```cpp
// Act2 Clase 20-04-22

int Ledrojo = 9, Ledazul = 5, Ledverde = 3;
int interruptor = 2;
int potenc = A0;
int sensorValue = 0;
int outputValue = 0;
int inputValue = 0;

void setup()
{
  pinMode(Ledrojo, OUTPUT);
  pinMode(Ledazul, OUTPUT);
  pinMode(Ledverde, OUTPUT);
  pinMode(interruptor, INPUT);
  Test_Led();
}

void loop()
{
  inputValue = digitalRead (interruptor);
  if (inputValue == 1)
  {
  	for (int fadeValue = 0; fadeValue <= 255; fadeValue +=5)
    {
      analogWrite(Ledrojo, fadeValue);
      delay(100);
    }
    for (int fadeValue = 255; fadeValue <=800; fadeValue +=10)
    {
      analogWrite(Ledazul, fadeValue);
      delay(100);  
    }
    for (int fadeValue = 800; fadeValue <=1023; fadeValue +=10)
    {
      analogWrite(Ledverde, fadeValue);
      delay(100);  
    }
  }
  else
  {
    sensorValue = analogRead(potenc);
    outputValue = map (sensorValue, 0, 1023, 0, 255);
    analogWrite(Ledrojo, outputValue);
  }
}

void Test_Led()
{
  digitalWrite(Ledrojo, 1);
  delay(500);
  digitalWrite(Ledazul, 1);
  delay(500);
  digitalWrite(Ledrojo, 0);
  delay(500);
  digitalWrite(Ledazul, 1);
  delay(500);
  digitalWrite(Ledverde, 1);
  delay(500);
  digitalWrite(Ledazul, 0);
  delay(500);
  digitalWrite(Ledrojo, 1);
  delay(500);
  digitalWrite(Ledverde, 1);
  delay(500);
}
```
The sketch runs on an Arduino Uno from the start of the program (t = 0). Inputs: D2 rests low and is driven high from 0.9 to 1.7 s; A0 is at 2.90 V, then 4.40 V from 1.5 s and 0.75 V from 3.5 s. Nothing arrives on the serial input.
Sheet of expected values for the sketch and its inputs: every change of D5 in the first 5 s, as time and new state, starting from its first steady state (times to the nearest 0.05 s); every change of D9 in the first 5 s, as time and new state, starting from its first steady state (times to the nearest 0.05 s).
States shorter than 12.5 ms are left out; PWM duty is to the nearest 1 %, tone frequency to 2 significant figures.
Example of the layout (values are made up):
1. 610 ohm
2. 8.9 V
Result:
1. 0 s low; 0.5 s high; 2.5 s low
2. 0 s high; 1 s low; 3 s high; 4 s PWM 15 %
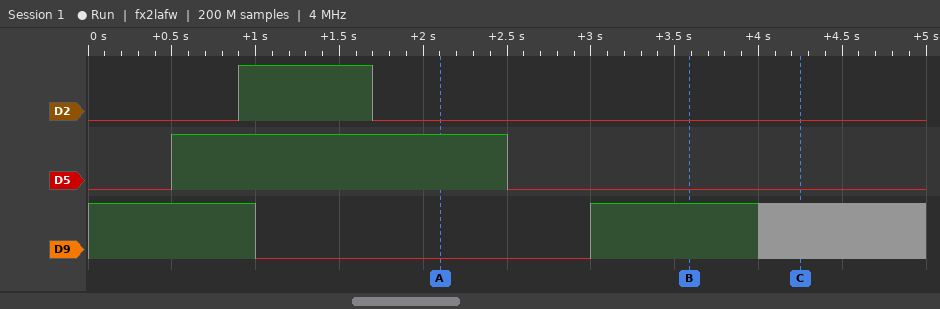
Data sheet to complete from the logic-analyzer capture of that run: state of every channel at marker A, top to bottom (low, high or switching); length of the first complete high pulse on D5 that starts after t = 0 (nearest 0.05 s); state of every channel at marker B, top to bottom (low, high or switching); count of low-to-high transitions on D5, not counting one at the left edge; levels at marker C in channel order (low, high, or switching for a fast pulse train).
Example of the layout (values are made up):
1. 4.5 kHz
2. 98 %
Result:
1. D2 low, D5 high, D9 low
2. 2.00 s
3. D2 low, D5 low, D9 high
4. 1
5. D2 low, D5 low, D9 switching
